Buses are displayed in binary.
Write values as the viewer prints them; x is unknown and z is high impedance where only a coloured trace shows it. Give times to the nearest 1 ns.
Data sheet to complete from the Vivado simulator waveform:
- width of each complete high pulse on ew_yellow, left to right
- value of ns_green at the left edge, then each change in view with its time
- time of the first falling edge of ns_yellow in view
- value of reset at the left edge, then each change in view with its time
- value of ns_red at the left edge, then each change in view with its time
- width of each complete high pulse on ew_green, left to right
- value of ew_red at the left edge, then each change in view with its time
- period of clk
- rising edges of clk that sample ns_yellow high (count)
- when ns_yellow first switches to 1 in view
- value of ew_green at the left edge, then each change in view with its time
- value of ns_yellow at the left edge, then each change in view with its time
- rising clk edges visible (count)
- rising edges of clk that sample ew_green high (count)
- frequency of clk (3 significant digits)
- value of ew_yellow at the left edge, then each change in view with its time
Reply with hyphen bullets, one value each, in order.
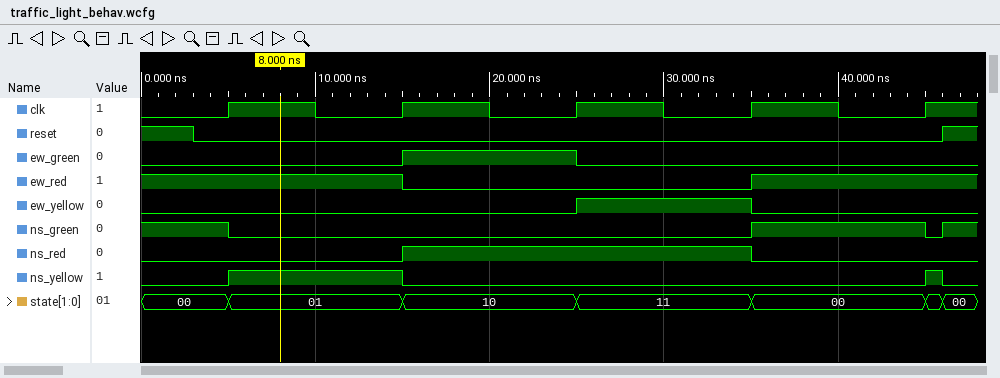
- 10 ns
- 1, 0 at 5 ns, 1 at 35 ns, 0 at 45 ns, 1 at 46 ns
- 15 ns
- 1, 0 at 3 ns, 1 at 46 ns
- 0, 1 at 15 ns, 0 at 35 ns
- 10 ns
- 1, 0 at 15 ns, 1 at 35 ns
- 10 ns
- 1
- 5 ns
- 0, 1 at 15 ns, 0 at 25 ns
- 0, 1 at 5 ns, 0 at 15 ns, 1 at 45 ns, 0 at 46 ns
- 5
- 1
- 100 MHz
- 0, 1 at 25 ns, 0 at 35 ns
